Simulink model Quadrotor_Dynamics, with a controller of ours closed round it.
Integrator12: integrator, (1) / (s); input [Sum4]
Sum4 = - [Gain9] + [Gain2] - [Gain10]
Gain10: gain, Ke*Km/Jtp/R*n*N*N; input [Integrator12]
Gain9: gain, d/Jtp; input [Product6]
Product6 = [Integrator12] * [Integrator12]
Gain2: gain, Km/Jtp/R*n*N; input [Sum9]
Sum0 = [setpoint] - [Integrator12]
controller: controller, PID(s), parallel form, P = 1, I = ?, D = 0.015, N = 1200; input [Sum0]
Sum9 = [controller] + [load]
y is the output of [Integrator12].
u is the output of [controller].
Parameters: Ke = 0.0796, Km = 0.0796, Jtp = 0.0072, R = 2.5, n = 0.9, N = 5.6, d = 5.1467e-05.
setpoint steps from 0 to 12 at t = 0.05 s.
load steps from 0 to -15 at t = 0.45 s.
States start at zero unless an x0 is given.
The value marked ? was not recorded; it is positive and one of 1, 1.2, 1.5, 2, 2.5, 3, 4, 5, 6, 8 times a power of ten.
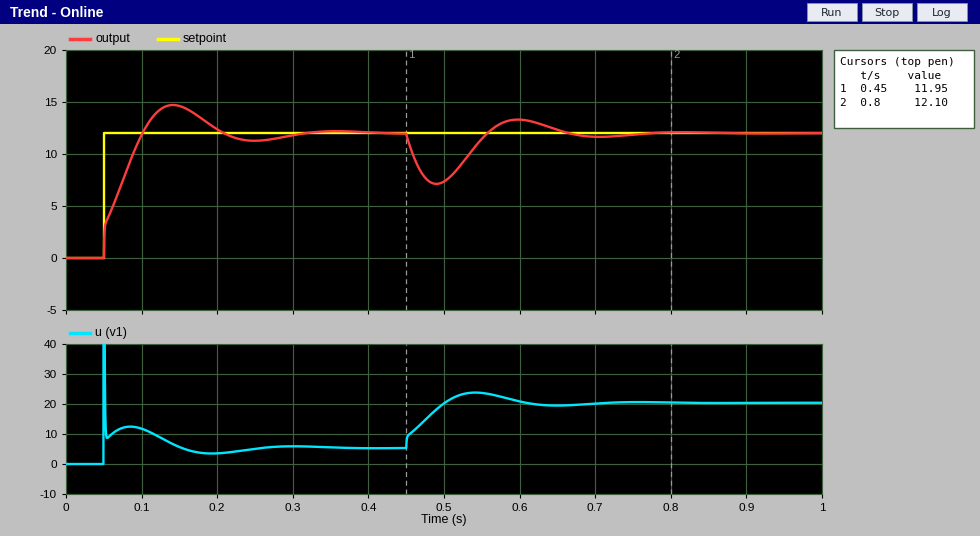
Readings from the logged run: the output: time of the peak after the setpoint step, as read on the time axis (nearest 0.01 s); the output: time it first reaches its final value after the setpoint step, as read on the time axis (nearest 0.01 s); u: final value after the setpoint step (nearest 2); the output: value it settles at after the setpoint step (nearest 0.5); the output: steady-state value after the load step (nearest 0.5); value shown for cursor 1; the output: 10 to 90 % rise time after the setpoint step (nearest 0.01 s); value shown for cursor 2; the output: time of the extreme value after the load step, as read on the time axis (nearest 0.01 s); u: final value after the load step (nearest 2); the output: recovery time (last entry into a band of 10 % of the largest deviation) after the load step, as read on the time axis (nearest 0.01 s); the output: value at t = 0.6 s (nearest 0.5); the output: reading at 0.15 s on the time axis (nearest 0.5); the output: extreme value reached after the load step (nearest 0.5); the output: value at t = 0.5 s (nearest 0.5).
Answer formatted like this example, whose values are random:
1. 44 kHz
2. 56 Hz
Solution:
1. 0.14 s
2. 0.10 s
3. 6
4. 12.0
5. 12.0
6. 11.95
7. 0.04 s
8. 12.10
9. 0.49 s
10. 20
11. 0.64 s
12. 13.5
13. 14.5
14. 7.0
15. 7.5
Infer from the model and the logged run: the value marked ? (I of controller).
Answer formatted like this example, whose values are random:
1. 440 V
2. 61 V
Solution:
1. 60
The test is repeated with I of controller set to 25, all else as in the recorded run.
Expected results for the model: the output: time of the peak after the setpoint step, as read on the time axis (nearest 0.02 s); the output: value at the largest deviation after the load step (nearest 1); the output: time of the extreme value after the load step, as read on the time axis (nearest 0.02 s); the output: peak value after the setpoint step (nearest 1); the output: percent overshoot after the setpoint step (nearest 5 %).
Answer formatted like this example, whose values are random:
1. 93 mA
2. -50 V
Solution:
1. 0.20 s
2. 6
3. 0.50 s
4. 13
5. 10 %
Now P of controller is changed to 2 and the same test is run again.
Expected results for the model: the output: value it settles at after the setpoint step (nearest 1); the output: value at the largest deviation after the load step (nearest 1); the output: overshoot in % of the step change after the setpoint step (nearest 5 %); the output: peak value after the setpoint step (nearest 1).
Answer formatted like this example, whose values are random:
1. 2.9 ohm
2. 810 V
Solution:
1. 12
2. 8
3. 10 %
4. 13
